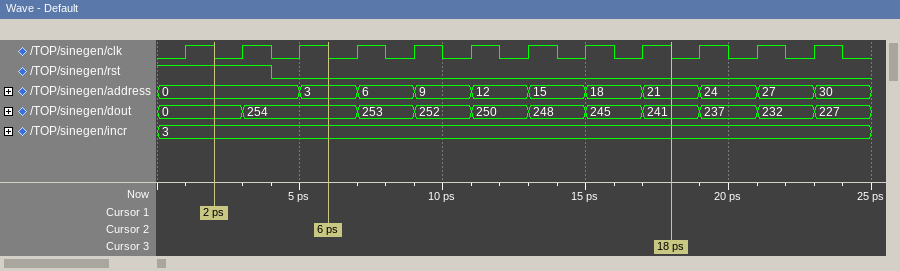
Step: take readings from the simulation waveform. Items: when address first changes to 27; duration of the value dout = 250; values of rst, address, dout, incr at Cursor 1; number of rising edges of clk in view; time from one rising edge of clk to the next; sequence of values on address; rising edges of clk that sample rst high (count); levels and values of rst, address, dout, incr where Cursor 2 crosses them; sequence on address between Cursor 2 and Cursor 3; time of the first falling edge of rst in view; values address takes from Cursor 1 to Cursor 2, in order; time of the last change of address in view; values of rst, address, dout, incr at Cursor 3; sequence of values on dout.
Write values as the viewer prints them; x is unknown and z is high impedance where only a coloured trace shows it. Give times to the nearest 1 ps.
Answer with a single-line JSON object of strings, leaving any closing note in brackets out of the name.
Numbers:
{"when address first changes to 27": "21 ps", "duration of the value dout = 250": "2 ps", "values of rst, address, dout, incr at Cursor 1": "rst=1, address=0, dout=0, incr=3", "number of rising edges of clk in view": "12", "time from one rising edge of clk to the next": "2 ps", "sequence of values on address": "0, 3, 6, 9, 12, 15, 18, 21, 24, 27, 30", "rising edges of clk that sample rst high": "2", "levels and values of rst, address, dout, incr where Cursor 2 crosses them": "rst=0, address=3, dout=254, incr=3", "sequence on address between Cursor 2 and Cursor 3": "3, 6, 9, 12, 15, 18, 21", "time of the first falling edge of rst in view": "4 ps", "values address takes from Cursor 1 to Cursor 2, in order": "0, 3", "time of the last change of address in view": "23 ps", "values of rst, address, dout, incr at Cursor 3": "rst=0, address=21, dout=241, incr=3", "sequence of values on dout": "0, 254, 253, 252, 250, 248, 245, 241, 237, 232, 227"}
